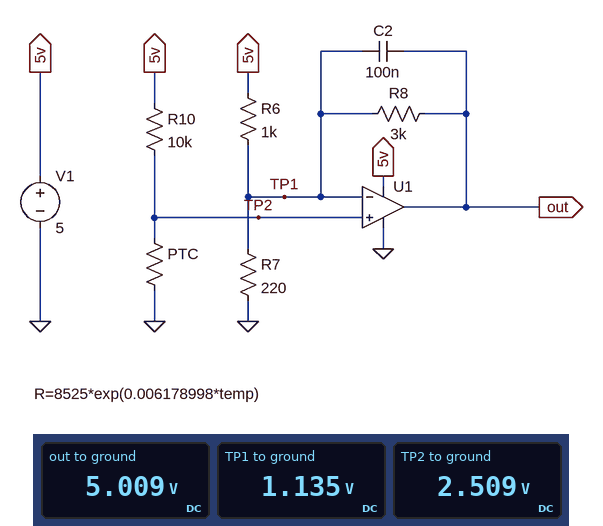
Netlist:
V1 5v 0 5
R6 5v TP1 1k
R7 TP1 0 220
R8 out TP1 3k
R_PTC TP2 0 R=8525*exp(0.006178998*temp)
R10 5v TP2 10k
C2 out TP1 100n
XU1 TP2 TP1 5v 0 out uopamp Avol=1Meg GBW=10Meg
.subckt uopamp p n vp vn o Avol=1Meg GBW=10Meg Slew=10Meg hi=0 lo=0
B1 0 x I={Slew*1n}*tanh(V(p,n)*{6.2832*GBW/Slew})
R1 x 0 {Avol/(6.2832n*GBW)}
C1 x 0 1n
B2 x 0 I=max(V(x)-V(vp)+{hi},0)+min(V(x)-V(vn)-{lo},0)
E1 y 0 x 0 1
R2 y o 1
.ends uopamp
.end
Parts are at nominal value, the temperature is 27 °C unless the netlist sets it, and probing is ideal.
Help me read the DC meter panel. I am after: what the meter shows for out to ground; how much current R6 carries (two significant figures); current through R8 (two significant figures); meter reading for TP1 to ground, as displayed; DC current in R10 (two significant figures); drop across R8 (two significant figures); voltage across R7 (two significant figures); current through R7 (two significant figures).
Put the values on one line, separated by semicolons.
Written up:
5.009 V; 3.9 mA; 1.3 mA; 1.135 V; 250 µA; 3.9 V; 1.1 V; 5.2 mA
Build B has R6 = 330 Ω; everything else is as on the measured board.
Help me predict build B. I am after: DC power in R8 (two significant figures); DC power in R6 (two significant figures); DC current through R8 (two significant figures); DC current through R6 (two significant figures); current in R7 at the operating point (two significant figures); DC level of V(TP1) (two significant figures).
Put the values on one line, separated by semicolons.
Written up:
2.8 mW; 25 mW; 960 µA; 8.7 mA; 9.7 mA; 2.1 V
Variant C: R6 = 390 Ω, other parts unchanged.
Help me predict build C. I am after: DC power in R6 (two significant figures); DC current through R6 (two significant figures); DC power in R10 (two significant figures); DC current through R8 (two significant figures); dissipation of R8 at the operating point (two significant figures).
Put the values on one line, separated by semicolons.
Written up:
24 mW; 7.8 mA; 620 µW; 1.0 mA; 3.1 mW
